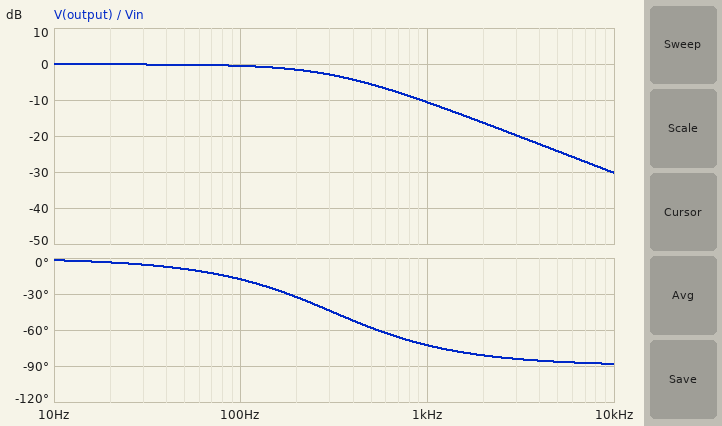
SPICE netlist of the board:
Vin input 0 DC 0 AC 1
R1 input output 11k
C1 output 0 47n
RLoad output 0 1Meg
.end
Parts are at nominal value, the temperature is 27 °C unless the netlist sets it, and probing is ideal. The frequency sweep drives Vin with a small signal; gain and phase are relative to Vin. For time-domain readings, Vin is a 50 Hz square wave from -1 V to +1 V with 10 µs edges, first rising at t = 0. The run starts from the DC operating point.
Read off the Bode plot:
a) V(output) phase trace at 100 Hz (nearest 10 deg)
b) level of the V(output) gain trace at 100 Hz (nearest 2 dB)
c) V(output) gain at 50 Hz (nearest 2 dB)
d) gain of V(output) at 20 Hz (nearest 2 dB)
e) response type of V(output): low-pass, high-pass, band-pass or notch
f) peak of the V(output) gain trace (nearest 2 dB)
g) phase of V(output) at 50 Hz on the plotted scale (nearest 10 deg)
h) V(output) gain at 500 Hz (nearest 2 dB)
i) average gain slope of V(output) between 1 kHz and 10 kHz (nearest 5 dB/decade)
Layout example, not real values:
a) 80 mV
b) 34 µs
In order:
a) -20 deg
b) 0 dB
c) 0 dB
d) 0 dB
e) low-pass
f) 0 dB
g) -10 deg
h) -6 dB
i) -20 dB/decade
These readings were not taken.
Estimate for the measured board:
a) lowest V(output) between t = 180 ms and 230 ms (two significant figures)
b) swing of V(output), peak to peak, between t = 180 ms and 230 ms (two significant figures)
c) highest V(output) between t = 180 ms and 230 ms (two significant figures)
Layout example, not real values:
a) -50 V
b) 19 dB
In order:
a) -990 mV
b) 2.0 V
c) 990 mV
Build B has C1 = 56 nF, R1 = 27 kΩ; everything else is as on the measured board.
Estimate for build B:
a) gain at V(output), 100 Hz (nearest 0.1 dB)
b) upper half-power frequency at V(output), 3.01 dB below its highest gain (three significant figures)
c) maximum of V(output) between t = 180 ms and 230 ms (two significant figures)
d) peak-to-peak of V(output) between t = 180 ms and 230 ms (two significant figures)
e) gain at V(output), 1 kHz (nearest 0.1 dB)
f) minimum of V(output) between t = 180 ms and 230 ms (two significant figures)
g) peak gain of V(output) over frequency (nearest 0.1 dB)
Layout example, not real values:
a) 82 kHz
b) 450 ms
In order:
a) -2.9 dB
b) 108 Hz
c) 970 mV
d) 1.9 V
e) -19.6 dB
f) -970 mV
g) -0.2 dB
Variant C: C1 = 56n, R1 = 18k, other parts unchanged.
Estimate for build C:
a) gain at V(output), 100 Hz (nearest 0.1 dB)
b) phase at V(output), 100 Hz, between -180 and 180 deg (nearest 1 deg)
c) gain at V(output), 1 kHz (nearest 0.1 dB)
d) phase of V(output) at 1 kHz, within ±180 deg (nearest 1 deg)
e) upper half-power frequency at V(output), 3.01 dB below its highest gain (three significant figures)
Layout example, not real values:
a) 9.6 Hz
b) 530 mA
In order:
a) -1.6 dB
b) -32 deg
c) -16.1 dB
d) -81 deg
e) 161 Hz
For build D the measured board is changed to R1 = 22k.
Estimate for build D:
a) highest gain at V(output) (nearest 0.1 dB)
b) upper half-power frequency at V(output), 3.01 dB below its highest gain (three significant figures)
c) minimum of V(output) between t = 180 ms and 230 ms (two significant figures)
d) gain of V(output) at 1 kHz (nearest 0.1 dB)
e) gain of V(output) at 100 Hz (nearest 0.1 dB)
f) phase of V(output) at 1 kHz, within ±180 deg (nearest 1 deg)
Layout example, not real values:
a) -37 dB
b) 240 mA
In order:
a) -0.2 dB
b) 157 Hz
c) -980 mV
d) -16.4 dB
e) -1.7 dB
f) -81 deg
